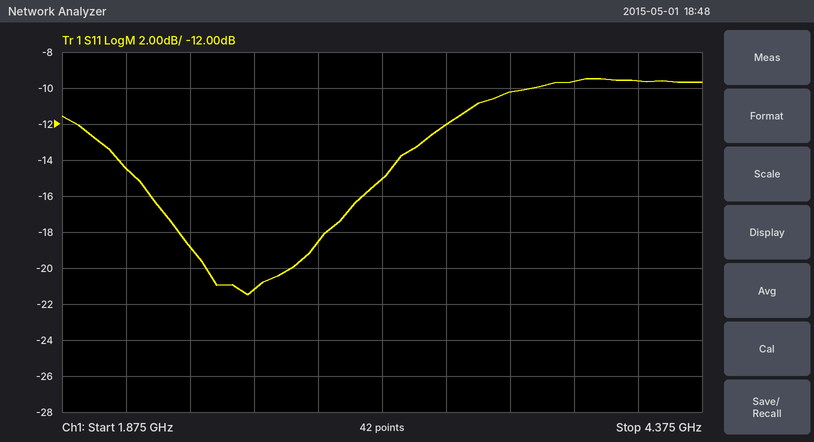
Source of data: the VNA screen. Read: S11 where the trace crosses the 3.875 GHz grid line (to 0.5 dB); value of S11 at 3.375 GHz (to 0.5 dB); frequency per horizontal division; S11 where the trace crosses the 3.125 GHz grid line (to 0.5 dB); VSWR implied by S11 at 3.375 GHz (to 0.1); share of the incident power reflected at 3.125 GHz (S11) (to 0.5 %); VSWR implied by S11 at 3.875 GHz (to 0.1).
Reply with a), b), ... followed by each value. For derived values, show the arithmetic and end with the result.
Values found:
a) -9.5 dB
b) -12.0 dB
c) 250 MHz
d) -15.0 dB
e) |Γ| = 10^(-12/20) = 0.2512; VSWR = (1 + 0.2512)/(1 − 0.2512) ≈ 1.7
f) 10^(-15/10) ≈ 3.16 %, so 3.0 % to the nearest 0.5 %
g) |Γ| = 10^(-9.5/20) = 0.3350; VSWR = (1 + 0.3350)/(1 − 0.3350) ≈ 2.0
